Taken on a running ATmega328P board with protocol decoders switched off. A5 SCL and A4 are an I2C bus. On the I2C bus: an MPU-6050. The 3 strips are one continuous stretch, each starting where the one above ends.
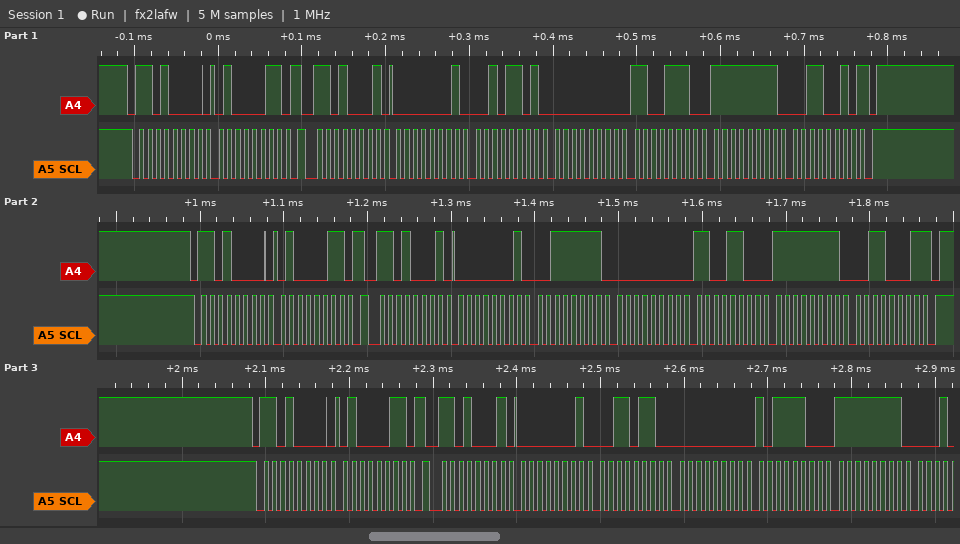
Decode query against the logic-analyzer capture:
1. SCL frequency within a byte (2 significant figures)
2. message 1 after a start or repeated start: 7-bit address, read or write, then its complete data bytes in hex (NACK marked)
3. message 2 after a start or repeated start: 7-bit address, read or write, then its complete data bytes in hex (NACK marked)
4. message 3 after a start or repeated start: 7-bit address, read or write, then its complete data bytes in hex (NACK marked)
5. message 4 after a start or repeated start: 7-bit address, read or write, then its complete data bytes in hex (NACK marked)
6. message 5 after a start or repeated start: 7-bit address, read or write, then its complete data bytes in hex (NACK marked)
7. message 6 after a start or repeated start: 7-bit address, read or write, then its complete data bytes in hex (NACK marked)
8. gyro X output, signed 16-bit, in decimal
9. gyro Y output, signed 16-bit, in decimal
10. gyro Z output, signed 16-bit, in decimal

100 kHz
0x68 write: 43
0x68 read: 01 2D 00 CE FF 32 NACK
0x68 write: 43
0x68 read: 01 3F 00 CC FF 31 NACK
0x68 write: 43
0x68 read: 01 36 00 BC FF
301
206
-206
